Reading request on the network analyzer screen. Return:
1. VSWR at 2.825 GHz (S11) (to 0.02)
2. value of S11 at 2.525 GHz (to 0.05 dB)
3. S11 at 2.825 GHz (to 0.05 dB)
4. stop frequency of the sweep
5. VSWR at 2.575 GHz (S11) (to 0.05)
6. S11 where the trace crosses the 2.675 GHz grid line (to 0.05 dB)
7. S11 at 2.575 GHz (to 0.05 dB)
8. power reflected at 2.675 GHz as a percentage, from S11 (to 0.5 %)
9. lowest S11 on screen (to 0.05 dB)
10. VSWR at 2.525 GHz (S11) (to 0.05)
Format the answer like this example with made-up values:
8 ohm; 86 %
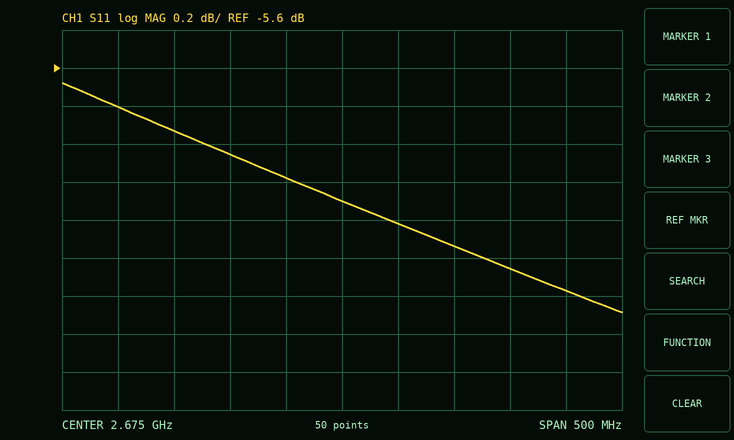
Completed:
2.74; -5.95 dB; -6.65 dB; 2.925 GHz; 3.00; -6.30 dB; -6.05 dB; 23.5 %; -6.90 dB; 3.05
